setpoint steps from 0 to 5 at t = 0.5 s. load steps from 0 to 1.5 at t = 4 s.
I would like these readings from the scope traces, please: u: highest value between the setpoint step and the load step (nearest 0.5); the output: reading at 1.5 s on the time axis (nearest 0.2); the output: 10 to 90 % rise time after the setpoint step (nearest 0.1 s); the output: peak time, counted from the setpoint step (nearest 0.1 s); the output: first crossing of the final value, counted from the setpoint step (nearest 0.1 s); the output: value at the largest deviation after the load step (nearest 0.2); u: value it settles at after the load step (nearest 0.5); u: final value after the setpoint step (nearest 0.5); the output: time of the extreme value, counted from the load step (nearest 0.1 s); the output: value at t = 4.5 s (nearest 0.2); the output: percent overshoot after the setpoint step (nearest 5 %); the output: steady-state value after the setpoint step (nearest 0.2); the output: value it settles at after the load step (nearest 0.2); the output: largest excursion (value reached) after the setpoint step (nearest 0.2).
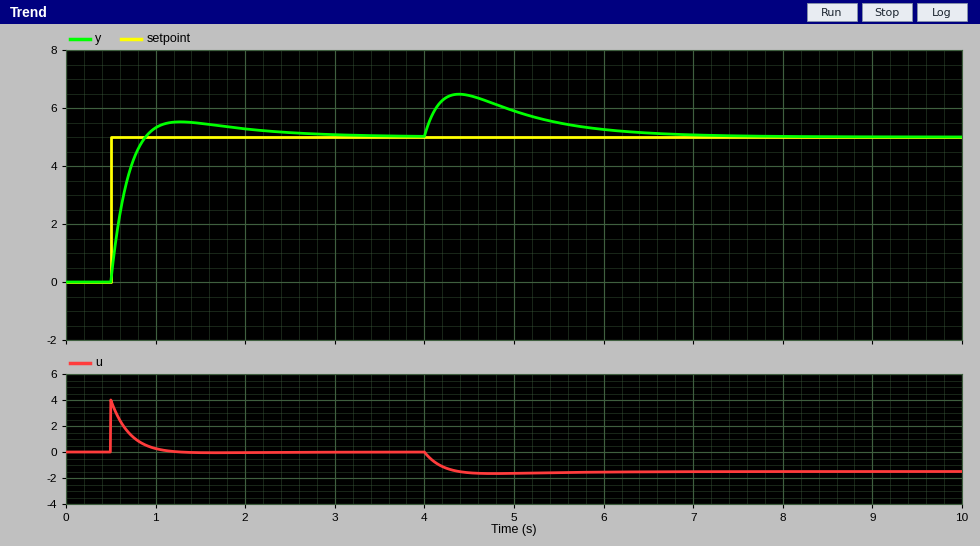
4.0
5.4
0.3 s
0.8 s
0.4 s
6.4
-1.5
0.0
0.4 s
6.4
10 %
5.0
5.0
5.6
